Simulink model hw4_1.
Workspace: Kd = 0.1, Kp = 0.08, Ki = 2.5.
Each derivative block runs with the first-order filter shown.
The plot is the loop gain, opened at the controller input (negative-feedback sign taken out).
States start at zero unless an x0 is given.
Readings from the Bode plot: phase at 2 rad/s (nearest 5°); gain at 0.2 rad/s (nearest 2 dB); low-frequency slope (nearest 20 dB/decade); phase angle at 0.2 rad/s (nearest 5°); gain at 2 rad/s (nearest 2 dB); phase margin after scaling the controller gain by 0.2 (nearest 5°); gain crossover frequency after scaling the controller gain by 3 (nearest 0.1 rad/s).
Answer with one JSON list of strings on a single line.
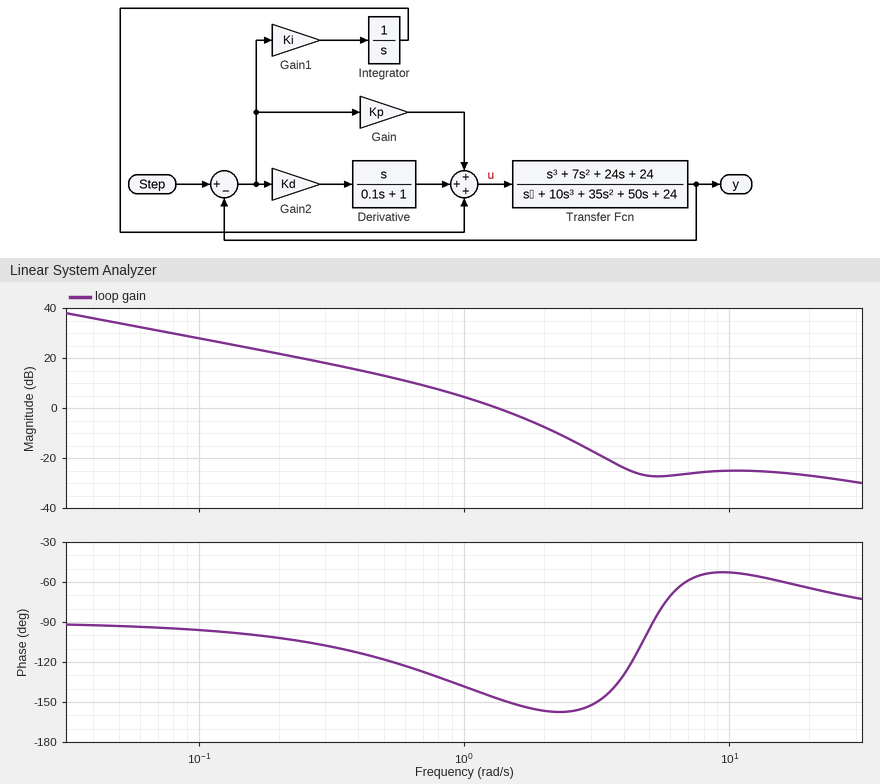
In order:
["-155°", "22 dB", "-20 dB/decade", "-100°", "-8 dB", "65°", "2.2 rad/s"]
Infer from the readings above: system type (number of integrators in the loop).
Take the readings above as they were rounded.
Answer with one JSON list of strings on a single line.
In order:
["1"]
